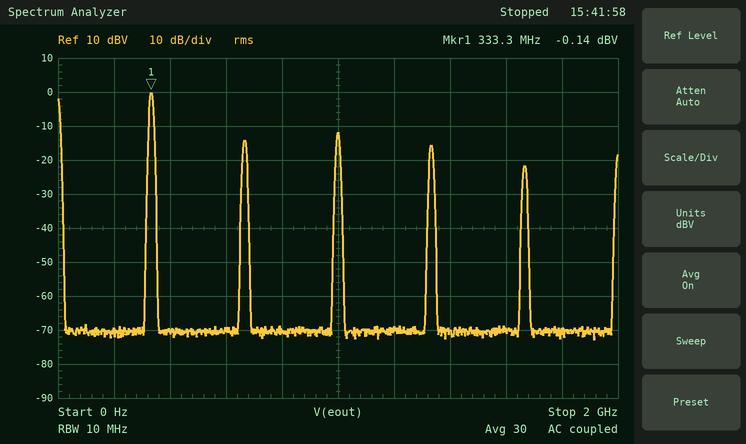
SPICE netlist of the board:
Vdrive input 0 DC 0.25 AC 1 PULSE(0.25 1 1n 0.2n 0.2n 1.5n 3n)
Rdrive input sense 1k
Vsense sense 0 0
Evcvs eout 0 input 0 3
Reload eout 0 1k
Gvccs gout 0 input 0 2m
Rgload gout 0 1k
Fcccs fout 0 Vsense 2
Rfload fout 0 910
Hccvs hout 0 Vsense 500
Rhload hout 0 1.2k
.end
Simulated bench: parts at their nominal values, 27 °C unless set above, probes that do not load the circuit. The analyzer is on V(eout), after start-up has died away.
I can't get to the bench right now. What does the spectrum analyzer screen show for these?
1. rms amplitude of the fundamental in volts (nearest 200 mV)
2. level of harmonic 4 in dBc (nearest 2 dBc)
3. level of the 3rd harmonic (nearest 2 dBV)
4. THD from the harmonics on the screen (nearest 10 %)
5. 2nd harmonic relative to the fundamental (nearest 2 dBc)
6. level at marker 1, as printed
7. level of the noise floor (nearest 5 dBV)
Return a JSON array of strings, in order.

["1.0 V", "-16 dBc", "-12 dBV", "40 %", "-14 dBc", "-0.14 dBV", "-70 dBV"]
